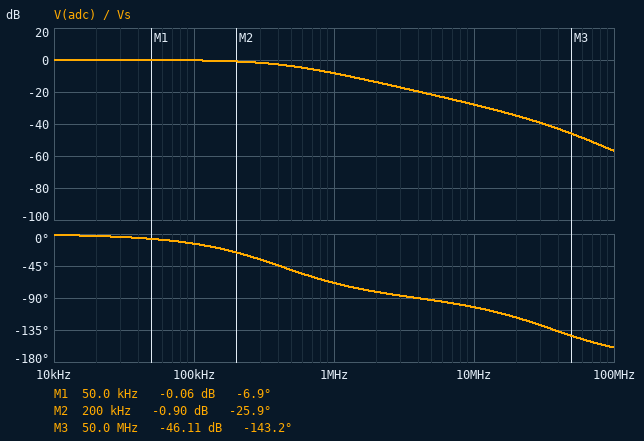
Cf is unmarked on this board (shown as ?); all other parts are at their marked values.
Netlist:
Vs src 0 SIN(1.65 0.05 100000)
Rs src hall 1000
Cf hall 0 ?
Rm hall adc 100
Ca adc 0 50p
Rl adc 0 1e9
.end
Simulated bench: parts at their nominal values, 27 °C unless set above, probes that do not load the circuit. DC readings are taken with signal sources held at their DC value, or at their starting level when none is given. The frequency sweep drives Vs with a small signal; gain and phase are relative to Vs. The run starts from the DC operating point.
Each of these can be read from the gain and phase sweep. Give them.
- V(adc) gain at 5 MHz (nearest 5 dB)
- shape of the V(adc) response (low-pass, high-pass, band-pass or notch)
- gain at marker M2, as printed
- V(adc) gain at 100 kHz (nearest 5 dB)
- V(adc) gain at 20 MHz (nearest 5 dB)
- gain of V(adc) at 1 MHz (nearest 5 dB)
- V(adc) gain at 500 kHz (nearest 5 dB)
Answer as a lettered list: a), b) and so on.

a) -20 dB
b) low-pass
c) -0.90 dB
d) 0 dB
e) -35 dB
f) -10 dB
g) -5 dB
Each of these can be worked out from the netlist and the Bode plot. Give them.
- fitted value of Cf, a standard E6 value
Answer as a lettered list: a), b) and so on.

a) 330 pF
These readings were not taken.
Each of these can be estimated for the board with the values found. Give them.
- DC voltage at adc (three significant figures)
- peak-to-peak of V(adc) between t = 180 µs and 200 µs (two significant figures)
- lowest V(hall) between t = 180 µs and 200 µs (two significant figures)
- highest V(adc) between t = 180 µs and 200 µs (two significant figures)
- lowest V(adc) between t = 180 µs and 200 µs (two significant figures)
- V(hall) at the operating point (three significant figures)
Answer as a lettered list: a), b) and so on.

a) 1.65 V
b) 97 mV
c) 1.6 V
d) 1.7 V
e) 1.6 V
f) 1.65 V
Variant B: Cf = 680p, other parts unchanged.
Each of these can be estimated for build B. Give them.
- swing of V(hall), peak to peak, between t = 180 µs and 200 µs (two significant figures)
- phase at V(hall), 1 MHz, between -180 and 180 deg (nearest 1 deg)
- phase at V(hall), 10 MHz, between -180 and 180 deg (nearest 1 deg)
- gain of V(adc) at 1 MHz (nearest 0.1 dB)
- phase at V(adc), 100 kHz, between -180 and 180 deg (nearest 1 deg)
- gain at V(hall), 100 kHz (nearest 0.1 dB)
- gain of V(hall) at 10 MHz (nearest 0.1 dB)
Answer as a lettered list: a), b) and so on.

a) 91 mV
b) -78 deg
c) -88 deg
d) -13.4 dB
e) -25 deg
f) -0.8 dB
g) -33.2 dB
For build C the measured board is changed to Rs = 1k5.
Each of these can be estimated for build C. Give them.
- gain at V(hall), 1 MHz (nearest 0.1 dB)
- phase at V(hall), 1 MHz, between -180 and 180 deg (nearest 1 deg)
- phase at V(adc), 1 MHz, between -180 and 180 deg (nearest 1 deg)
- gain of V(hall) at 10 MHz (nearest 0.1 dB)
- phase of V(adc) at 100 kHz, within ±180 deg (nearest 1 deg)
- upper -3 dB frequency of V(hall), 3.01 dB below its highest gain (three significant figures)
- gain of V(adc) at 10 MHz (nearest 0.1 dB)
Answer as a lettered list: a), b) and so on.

a) -11.4 dB
b) -74 deg
c) -76 deg
d) -31.0 dB
e) -20 deg
f) 279 kHz
g) -31.4 dB
